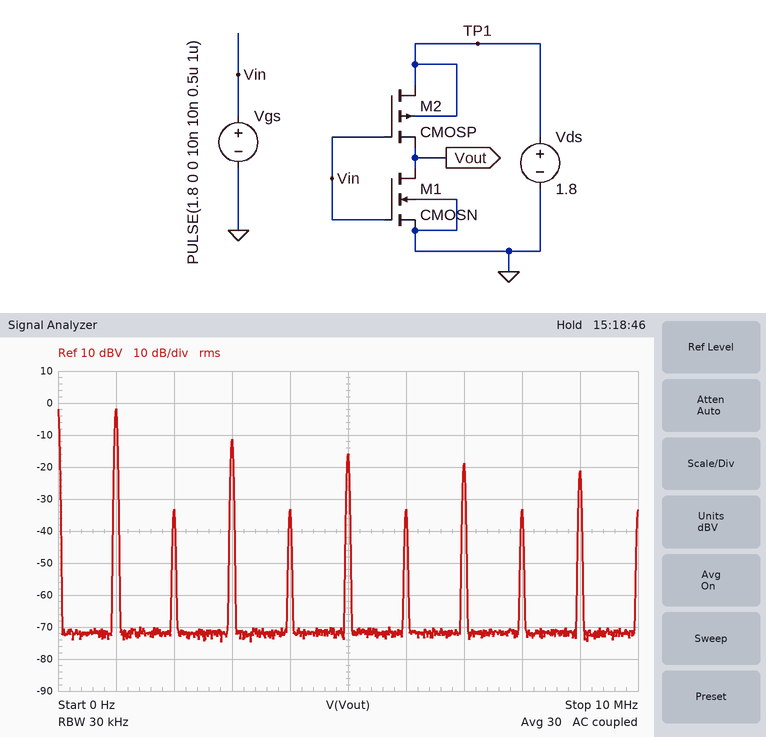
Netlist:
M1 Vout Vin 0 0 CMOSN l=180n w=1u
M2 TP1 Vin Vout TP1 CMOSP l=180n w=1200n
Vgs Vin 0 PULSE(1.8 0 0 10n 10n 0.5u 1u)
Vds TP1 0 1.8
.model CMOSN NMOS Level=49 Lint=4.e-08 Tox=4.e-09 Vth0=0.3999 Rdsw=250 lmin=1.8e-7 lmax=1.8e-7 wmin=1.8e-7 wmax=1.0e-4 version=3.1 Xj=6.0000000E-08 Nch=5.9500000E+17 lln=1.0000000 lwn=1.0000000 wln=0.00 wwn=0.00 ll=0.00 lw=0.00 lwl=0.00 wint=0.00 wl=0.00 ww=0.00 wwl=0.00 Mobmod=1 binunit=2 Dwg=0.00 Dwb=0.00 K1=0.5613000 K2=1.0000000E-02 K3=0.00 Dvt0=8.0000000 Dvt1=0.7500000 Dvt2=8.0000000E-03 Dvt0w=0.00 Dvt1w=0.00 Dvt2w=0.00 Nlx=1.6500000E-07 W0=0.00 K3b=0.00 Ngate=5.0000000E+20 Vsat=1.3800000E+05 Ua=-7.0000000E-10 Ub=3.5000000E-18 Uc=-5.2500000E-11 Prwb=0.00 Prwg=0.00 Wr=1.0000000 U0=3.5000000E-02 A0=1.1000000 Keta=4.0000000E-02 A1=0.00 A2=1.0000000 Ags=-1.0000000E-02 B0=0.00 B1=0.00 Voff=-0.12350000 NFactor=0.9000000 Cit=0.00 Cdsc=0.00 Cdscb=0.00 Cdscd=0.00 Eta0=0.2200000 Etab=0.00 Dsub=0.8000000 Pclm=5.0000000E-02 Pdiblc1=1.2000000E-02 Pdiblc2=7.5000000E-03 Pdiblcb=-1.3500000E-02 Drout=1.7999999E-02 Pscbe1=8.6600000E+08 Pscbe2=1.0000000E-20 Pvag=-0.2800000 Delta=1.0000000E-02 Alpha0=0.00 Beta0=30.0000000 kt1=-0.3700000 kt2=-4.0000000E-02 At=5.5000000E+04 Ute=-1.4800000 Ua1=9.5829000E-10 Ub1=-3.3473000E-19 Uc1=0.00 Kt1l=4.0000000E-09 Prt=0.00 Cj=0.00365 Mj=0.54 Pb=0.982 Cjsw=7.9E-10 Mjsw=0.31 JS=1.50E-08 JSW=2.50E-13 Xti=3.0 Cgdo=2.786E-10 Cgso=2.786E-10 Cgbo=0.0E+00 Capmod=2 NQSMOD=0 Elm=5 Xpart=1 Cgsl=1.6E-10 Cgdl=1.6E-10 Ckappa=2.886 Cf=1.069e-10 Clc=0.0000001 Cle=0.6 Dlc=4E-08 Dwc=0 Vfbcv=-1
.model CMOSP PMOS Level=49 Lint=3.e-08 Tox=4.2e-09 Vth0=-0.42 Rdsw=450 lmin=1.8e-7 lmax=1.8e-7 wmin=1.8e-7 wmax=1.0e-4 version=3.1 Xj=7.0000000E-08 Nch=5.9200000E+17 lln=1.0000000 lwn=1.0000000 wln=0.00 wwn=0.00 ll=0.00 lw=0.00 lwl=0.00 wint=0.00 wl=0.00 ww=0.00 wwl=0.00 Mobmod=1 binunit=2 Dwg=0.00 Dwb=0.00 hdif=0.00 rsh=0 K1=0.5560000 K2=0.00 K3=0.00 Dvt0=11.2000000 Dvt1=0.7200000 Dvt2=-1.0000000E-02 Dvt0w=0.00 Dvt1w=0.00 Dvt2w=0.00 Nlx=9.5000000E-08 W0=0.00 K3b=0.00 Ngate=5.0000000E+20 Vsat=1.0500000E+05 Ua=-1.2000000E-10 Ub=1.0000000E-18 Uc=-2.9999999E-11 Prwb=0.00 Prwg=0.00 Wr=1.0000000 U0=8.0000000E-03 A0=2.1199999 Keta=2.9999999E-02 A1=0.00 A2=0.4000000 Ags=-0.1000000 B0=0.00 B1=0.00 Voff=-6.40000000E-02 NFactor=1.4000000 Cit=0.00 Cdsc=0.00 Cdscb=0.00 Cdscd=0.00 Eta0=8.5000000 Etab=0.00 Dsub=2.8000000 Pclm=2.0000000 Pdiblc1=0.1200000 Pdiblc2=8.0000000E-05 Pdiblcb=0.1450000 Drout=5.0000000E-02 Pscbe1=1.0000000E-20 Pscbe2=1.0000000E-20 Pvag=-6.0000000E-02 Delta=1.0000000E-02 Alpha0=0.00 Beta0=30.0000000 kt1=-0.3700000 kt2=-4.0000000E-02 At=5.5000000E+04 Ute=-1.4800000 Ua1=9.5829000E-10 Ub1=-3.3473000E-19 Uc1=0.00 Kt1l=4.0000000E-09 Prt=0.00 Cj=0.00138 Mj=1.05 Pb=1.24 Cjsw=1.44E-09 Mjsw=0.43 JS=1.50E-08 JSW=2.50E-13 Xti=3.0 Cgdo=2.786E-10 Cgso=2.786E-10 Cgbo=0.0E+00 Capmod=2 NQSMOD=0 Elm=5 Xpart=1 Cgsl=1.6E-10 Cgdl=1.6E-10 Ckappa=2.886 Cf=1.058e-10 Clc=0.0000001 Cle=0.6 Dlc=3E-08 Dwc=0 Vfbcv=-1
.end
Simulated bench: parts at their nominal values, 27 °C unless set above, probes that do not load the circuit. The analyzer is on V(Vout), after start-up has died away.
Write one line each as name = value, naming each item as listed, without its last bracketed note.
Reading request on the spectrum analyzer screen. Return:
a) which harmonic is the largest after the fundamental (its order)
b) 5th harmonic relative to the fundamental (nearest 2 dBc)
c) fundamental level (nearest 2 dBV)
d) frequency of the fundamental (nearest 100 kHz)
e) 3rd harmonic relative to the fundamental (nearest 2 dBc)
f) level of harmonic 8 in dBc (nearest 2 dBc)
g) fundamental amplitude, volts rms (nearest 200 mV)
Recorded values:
which harmonic is the largest after the fundamental = 3
5th harmonic relative to the fundamental = -14 dBc
fundamental level = -2 dBV
frequency of the fundamental = 1.0 MHz
3rd harmonic relative to the fundamental = -10 dBc
level of harmonic 8 in dBc = -32 dBc
fundamental amplitude, volts rms = 800 mV
